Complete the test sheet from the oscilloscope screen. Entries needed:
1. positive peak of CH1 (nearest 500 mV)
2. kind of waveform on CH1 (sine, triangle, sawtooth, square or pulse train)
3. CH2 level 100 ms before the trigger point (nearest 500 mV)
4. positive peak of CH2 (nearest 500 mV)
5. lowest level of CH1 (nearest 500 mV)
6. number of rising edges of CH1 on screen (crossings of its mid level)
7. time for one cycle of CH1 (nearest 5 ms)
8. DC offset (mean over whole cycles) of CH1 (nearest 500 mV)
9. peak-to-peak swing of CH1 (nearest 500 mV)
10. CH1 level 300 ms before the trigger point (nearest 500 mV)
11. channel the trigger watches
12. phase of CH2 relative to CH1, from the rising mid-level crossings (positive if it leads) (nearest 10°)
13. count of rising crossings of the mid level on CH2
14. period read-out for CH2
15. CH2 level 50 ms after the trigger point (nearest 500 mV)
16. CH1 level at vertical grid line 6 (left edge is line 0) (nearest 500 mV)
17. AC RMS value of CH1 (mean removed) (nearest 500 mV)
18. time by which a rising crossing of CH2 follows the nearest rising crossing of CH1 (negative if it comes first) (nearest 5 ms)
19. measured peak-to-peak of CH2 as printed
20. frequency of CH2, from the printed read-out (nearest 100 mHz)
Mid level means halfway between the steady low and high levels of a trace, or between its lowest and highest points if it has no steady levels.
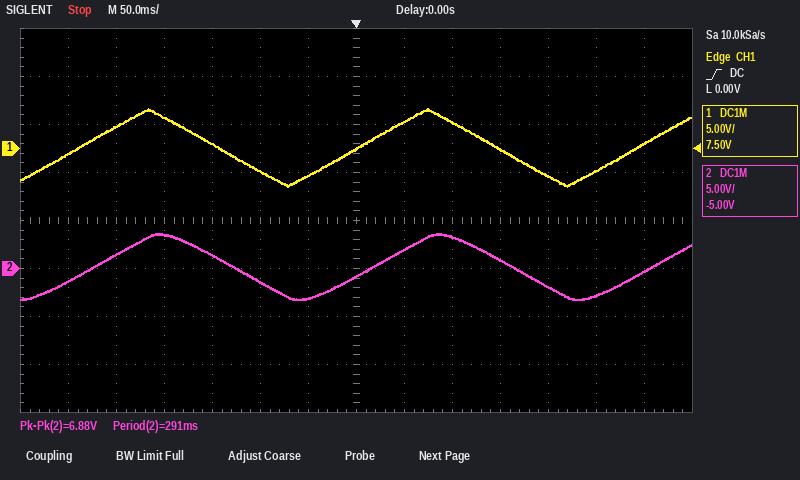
4.0 V
triangle
-1.5 V
3.5 V
-4.0 V
3
290 ms
0.0 V
8.0 V
-500 mV
CH1
-20°
3
291 ms
2.0 V
-3.0 V
2.5 V
+15 ms
6.88 V
3.4 Hz
